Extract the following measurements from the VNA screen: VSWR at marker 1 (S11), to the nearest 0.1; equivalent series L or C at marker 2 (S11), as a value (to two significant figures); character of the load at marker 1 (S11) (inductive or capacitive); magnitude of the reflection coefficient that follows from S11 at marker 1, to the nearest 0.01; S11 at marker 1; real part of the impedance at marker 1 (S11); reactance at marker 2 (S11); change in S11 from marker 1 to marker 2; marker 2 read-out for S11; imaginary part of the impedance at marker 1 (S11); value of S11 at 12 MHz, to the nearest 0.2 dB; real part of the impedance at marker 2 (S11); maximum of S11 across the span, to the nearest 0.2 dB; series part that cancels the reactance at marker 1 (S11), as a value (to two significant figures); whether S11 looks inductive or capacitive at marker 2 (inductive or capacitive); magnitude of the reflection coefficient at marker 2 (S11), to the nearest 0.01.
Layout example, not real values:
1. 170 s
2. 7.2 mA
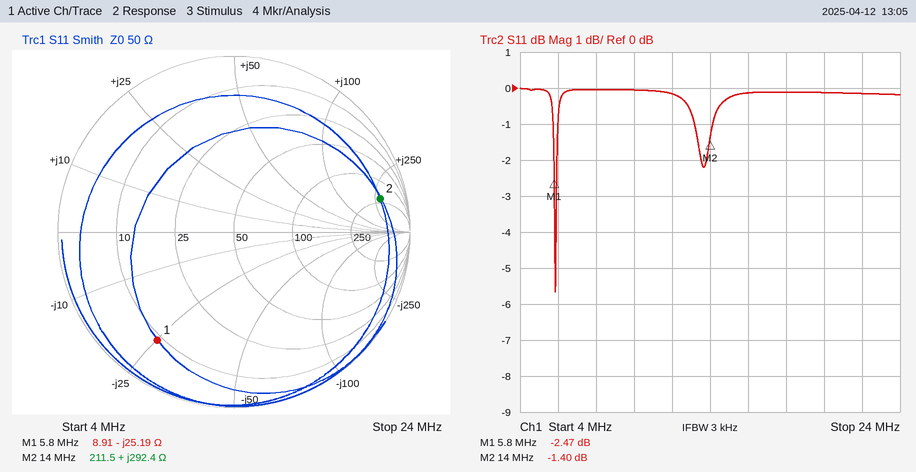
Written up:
1. 7.1
2. 3.3 µH
3. capacitive
4. 0.75
5. -2.47 dB
6. 8.91 Ω
7. +292.4 Ω
8. 1.07 dB
9. -1.40 dB
10. -25.19 Ω
11. -0.2 dB
12. 211.5 Ω
13. 0.0 dB
14. 690 nH
15. inductive
16. 0.85
